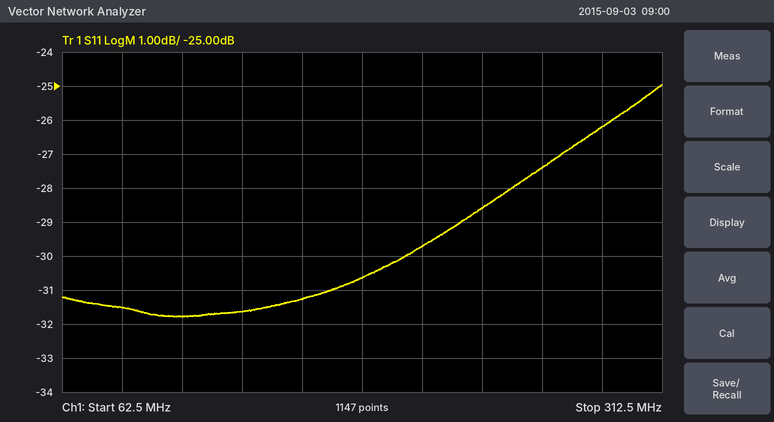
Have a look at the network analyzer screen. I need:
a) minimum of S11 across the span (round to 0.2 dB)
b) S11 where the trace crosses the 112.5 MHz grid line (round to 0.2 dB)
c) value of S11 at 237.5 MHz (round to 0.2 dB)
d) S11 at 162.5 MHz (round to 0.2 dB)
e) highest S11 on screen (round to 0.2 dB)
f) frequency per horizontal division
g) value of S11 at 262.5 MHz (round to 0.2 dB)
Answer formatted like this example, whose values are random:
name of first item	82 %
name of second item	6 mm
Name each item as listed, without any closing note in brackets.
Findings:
minimum of S11 across the span	-31.8 dB
S11 where the trace crosses the 112.5 MHz grid line	-31.8 dB
value of S11 at 237.5 MHz	-28.6 dB
S11 at 162.5 MHz	-31.2 dB
highest S11 on screen	-25.0 dB
frequency per horizontal division	25 MHz
value of S11 at 262.5 MHz	-27.4 dB
